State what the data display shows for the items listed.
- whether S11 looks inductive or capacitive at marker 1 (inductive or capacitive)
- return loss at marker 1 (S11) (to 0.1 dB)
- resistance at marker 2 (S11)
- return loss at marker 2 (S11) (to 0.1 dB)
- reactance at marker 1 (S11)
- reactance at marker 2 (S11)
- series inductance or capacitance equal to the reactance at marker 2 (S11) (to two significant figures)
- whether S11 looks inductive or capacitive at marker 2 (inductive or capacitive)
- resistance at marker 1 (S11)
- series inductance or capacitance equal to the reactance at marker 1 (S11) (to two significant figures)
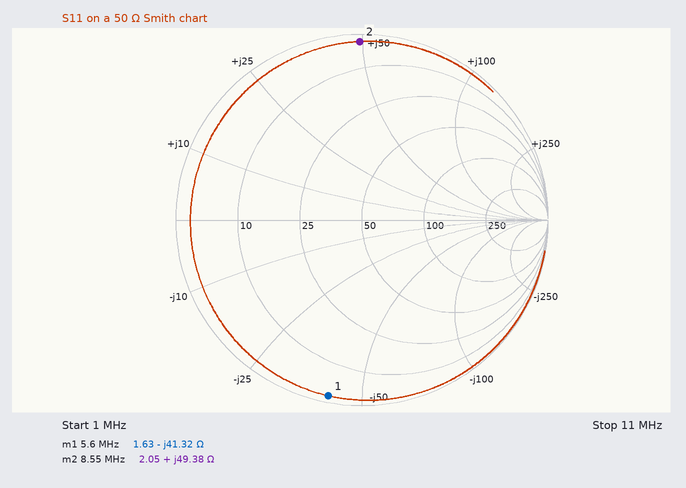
capacitive
0.3 dB
2.05 Ω
0.4 dB
-41.32 Ω
+49.38 Ω
920 nH
inductive
1.63 Ω
690 pF
